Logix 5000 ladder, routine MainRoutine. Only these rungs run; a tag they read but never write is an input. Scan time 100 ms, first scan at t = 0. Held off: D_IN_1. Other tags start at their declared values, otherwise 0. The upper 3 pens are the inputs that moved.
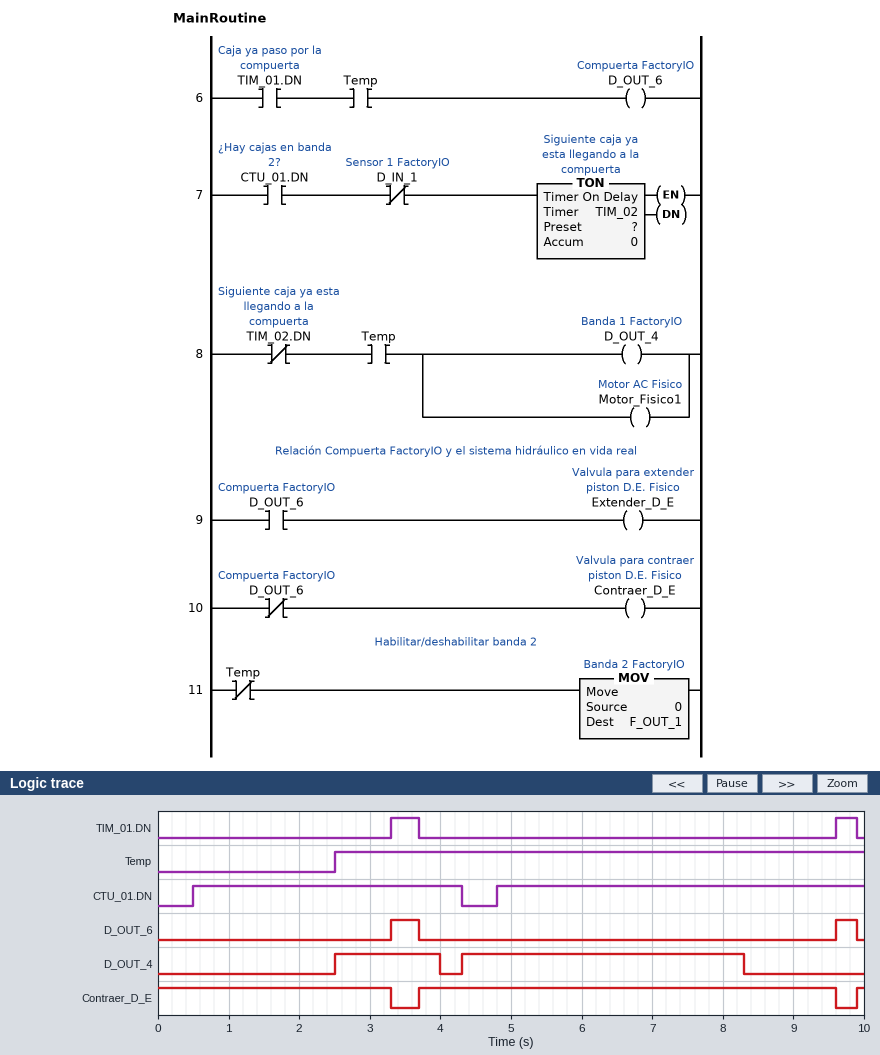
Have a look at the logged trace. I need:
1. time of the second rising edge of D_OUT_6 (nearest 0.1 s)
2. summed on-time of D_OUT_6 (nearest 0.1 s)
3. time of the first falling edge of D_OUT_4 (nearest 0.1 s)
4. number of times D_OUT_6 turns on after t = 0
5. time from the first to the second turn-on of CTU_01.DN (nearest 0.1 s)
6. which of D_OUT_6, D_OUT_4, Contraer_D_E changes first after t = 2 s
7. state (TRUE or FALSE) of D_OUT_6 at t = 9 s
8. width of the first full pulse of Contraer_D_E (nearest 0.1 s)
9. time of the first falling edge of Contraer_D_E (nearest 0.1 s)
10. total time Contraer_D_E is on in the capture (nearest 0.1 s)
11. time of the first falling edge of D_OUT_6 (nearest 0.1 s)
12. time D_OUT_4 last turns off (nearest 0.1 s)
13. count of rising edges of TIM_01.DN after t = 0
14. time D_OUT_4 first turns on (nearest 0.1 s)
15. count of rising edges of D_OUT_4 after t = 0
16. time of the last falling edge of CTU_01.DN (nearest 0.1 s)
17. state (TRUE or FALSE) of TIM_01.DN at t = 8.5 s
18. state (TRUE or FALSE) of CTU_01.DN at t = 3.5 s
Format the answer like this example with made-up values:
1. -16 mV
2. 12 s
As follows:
1. 9.6 s
2. 0.7 s
3. 4.0 s
4. 2
5. 4.3 s
6. D_OUT_4
7. FALSE
8. 5.9 s
9. 3.3 s
10. 9.3 s
11. 3.7 s
12. 8.3 s
13. 2
14. 2.5 s
15. 2
16. 4.3 s
17. FALSE
18. TRUE
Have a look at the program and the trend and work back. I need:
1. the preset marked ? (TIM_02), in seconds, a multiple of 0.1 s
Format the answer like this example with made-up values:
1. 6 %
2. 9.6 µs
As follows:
1. 3.5 s
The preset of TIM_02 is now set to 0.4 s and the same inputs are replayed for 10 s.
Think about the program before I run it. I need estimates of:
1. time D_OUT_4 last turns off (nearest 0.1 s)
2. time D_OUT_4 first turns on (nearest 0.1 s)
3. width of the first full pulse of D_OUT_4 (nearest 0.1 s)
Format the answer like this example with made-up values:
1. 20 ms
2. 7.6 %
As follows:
1. 5.2 s
2. 4.3 s
3. 0.9 s
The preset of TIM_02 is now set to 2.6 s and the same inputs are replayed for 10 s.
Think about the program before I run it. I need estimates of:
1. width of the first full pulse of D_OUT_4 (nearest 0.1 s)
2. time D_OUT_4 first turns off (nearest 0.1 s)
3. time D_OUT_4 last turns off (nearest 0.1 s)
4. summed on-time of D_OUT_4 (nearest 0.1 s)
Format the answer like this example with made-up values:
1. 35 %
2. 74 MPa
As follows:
1. 0.6 s
2. 3.1 s
3. 7.4 s
4. 3.7 s
